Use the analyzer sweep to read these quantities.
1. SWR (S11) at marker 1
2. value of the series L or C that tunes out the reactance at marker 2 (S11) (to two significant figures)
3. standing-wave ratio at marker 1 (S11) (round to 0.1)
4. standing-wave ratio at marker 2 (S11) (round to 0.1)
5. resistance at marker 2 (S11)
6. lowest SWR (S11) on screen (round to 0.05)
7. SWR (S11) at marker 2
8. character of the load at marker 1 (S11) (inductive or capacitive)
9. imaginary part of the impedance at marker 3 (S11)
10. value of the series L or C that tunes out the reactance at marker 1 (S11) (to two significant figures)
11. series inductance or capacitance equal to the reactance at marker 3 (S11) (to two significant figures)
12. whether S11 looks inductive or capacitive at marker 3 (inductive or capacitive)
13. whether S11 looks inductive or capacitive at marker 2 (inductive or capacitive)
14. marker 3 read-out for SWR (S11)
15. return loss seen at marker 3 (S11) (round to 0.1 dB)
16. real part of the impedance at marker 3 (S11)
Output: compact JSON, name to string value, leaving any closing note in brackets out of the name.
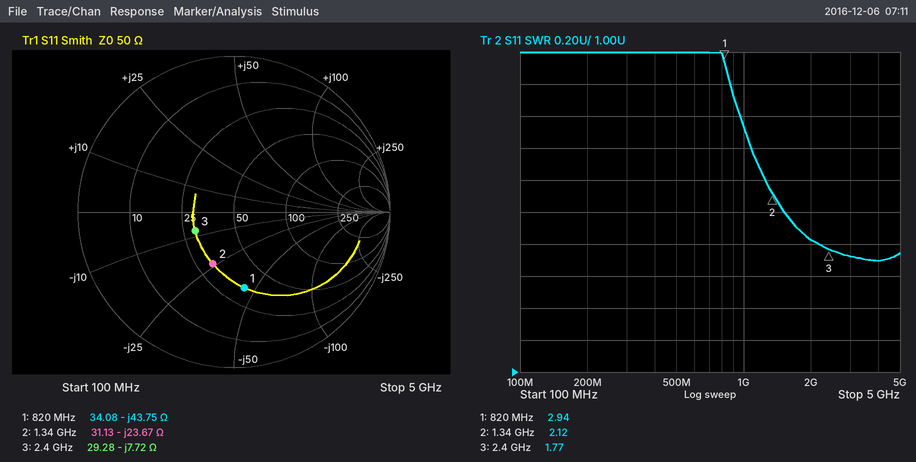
{"SWR (S11) at marker 1": "2.94", "value of the series L or C that tunes out the reactance at marker 2 (S11)": "2.8 nH", "standing-wave ratio at marker 1 (S11)": "2.9", "standing-wave ratio at marker 2 (S11)": "2.1", "resistance at marker 2": "31.13 Ω", "lowest SWR (S11) on screen": "1.70", "SWR (S11) at marker 2": "2.12", "character of the load at marker 1 (S11)": "capacitive", "imaginary part of the impedance at marker 3": "-7.72 Ω", "value of the series L or C that tunes out the reactance at marker 1 (S11)": "8.5 nH", "series inductance or capacitance equal to the reactance at marker 3 (S11)": "8.6 pF", "whether S11 looks inductive or capacitive at marker 3": "capacitive", "whether S11 looks inductive or capacitive at marker 2": "capacitive", "marker 3 read-out for SWR": "1.77", "return loss seen at marker 3 (S11)": "11.1 dB", "real part of the impedance at marker 3": "29.28 Ω"}
